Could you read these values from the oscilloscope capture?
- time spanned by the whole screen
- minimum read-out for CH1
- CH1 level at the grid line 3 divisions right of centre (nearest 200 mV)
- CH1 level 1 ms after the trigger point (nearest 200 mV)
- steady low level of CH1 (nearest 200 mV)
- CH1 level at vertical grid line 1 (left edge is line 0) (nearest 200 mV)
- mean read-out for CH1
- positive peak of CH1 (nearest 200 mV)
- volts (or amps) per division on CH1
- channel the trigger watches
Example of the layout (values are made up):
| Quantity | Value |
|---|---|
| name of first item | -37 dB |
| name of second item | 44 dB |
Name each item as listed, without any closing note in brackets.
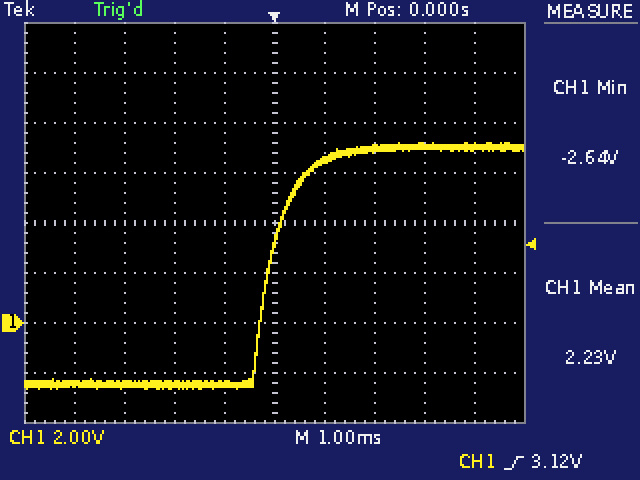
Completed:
| Quantity | Value |
|---|---|
| time spanned by the whole screen | 10 ms |
| minimum read-out for CH1 | -2.64 V |
| CH1 level at the grid line 3 divisions right of centre | 7.0 V |
| CH1 level 1 ms after the trigger point | 6.4 V |
| steady low level of CH1 | -2.4 V |
| CH1 level at vertical grid line 1 (left edge is line 0) | -2.4 V |
| mean read-out for CH1 | 2.23 V |
| positive peak of CH1 | 7.2 V |
| volts (or amps) per division on CH1 | 2 V |
| channel the trigger watches | CH1 |
